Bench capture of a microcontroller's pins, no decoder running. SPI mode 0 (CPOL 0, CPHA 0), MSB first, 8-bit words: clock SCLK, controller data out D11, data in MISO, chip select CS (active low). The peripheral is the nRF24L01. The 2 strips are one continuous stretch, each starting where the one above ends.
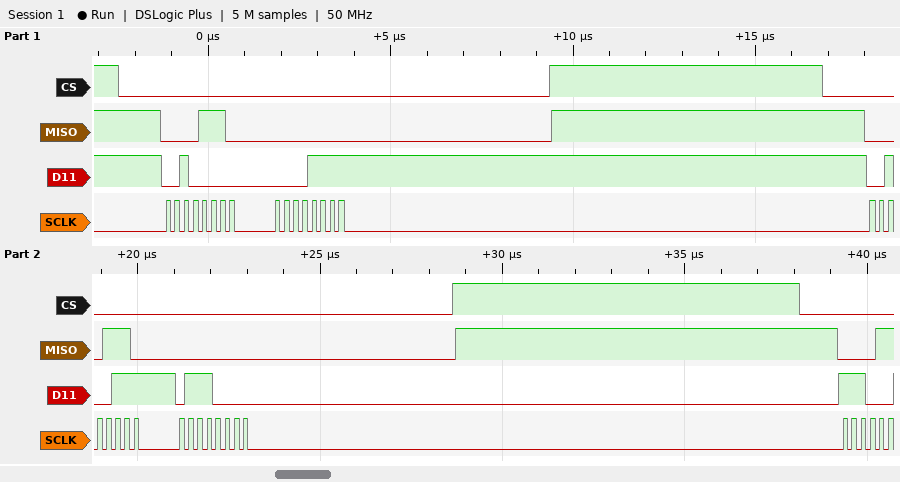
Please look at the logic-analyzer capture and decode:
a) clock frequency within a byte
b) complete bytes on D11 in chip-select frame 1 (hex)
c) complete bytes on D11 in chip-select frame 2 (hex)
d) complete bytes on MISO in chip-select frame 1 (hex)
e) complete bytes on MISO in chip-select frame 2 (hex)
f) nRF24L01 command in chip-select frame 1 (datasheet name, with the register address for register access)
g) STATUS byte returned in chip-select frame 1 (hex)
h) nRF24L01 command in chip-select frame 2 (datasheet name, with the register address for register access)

4 MHz
20 0F
27 70
0E 00
0E 00
W_REGISTER 0x00
0x0E
W_REGISTER 0x07
